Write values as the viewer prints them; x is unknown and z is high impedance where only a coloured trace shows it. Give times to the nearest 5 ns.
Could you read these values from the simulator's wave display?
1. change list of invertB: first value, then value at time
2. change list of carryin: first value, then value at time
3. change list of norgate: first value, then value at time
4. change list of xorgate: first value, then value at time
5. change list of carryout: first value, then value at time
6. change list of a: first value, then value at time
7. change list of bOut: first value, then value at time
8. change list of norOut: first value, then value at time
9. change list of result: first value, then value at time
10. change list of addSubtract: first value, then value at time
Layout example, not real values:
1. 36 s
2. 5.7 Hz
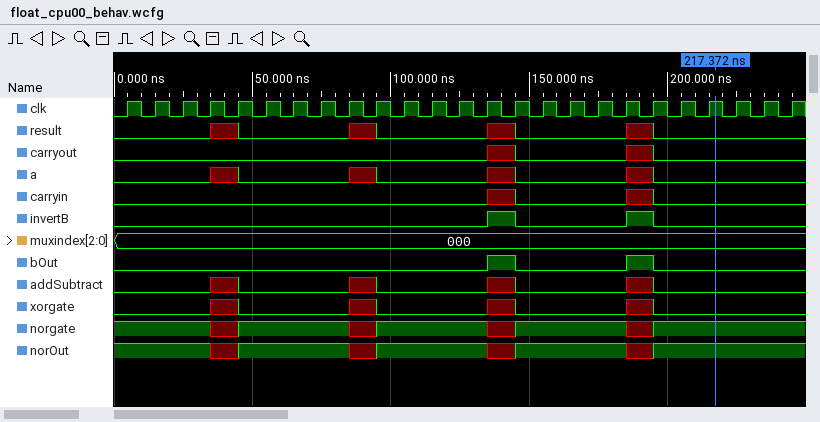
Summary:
1. 0, 1 at 135 ns, 0 at 145 ns, 1 at 185 ns, 0 at 195 ns
2. 0, x at 135 ns, 0 at 145 ns, x at 185 ns, 0 at 195 ns
3. 1, x at 35 ns, 1 at 45 ns, x at 85 ns, 1 at 95 ns, x at 135 ns, 1 at 145 ns, x at 185 ns, 1 at 195 ns
4. 0, x at 35 ns, 0 at 45 ns, x at 85 ns, 0 at 95 ns, x at 135 ns, 0 at 145 ns, x at 185 ns, 0 at 195 ns
5. 0, x at 135 ns, 0 at 145 ns, x at 185 ns, 0 at 195 ns
6. 0, x at 35 ns, 0 at 45 ns, x at 85 ns, 0 at 95 ns, x at 135 ns, 0 at 145 ns, x at 185 ns, 0 at 195 ns
7. 0, 1 at 135 ns, 0 at 145 ns, 1 at 185 ns, 0 at 195 ns
8. 1, x at 35 ns, 1 at 45 ns, x at 85 ns, 1 at 95 ns, x at 135 ns, 1 at 145 ns, x at 185 ns, 1 at 195 ns
9. 0, x at 35 ns, 0 at 45 ns, x at 85 ns, 0 at 95 ns, x at 135 ns, 0 at 145 ns, x at 185 ns, 0 at 195 ns
10. 0, x at 35 ns, 0 at 45 ns, x at 85 ns, 0 at 95 ns, x at 135 ns, 0 at 145 ns, x at 185 ns, 0 at 195 ns
